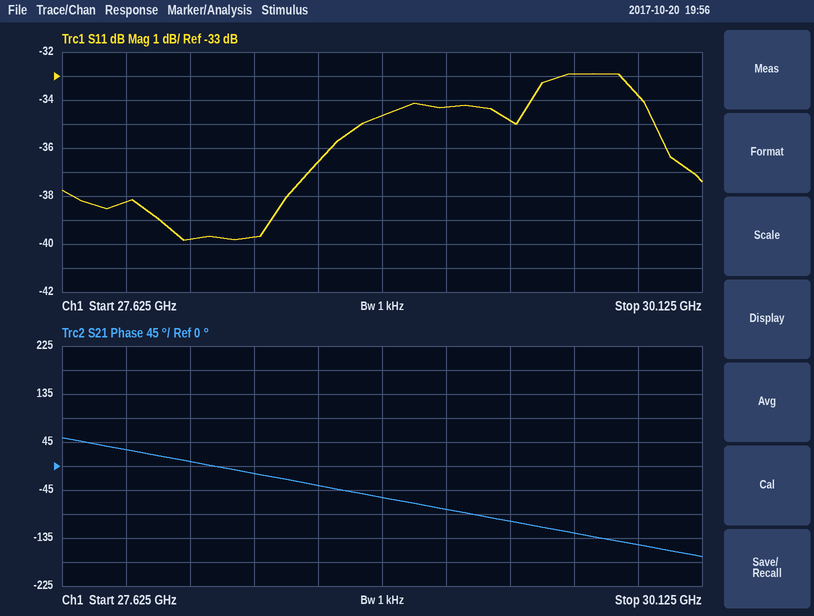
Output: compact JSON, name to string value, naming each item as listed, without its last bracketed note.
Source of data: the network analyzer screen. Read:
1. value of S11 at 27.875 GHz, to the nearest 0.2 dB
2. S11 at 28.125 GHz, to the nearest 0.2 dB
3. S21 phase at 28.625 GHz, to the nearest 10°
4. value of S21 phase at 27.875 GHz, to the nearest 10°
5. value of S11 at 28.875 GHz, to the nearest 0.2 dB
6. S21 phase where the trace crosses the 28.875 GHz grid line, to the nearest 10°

{"value of S11 at 27.875 GHz, to the nearest 0.2 dB": "-38.2 dB", "S11 at 28.125 GHz, to the nearest 0.2 dB": "-39.8 dB", "S21 phase at 28.625 GHz, to the nearest 10°": "-40°", "value of S21 phase at 27.875 GHz, to the nearest 10°": "30°", "value of S11 at 28.875 GHz, to the nearest 0.2 dB": "-34.6 dB", "S21 phase where the trace crosses the 28.875 GHz grid line, to the nearest 10°": "-60°"}
